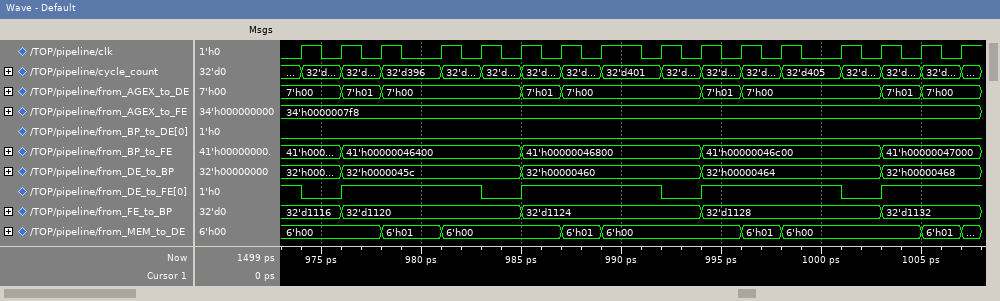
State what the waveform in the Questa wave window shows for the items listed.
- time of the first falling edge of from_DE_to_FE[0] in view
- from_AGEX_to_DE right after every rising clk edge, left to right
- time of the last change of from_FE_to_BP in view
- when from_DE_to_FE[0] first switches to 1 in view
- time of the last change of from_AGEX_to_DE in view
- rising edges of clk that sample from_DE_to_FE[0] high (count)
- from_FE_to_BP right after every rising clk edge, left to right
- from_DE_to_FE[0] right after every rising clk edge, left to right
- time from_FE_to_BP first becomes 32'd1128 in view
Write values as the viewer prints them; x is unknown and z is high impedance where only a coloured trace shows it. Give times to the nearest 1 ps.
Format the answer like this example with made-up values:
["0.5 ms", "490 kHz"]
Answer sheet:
["974 ps", "7'h00, 7'h01, 7'h00, 7'h00, 7'h00, 7'h01, 7'h00, 7'h00, 7'h00, 7'h01, 7'h00, 7'h00, 7'h00, 7'h01, 7'h00, 7'h00", "1003 ps", "976 ps", "1005 ps", "12", "32'd1116, 32'd1120, 32'd1120, 32'd1120, 32'd1120, 32'd1124, 32'd1124, 32'd1124, 32'd1124, 32'd1128, 32'd1128, 32'd1128, 32'd1128, 32'd1132, 32'd1132, 32'd1132", "0 1 1 1 0 1 1 1 0 1 1 1 0 1 1 1", "994 ps"]
